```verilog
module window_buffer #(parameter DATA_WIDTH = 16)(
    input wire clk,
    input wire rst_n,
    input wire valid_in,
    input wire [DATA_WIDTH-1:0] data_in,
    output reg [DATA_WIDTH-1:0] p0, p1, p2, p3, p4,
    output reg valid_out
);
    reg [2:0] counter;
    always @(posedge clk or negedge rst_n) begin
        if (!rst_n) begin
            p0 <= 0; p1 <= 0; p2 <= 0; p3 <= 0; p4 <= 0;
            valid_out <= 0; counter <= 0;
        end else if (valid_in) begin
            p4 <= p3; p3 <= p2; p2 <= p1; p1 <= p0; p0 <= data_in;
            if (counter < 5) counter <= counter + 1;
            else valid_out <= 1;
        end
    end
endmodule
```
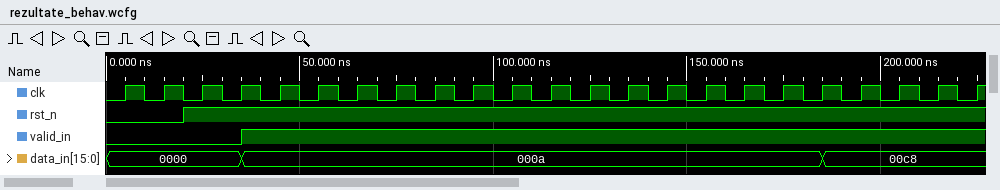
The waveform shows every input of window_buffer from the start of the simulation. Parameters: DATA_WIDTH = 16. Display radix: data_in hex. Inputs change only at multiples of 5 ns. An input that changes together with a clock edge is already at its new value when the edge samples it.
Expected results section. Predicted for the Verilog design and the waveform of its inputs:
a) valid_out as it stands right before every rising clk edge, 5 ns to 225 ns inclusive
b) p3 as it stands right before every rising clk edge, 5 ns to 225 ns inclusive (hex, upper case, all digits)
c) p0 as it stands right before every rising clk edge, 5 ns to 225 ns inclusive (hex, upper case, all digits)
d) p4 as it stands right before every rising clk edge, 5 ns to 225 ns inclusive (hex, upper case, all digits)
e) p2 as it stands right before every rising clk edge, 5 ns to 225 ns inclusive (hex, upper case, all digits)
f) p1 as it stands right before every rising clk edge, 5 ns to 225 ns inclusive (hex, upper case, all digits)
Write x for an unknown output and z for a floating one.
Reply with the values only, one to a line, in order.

0 0 0 0 0 0 0 0 0 1 1 1 1 1 1 1 1 1 1 1 1 1 1
0000, 0000, 0000, 0000, 0000, 0000, 0000, 000A, 000A, 000A, 000A, 000A, 000A, 000A, 000A, 000A, 000A, 000A, 000A, 000A, 000A, 000A, 00C8
0000, 0000, 0000, 0000, 000A, 000A, 000A, 000A, 000A, 000A, 000A, 000A, 000A, 000A, 000A, 000A, 000A, 000A, 000A, 00C8, 00C8, 00C8, 00C8
0000, 0000, 0000, 0000, 0000, 0000, 0000, 0000, 000A, 000A, 000A, 000A, 000A, 000A, 000A, 000A, 000A, 000A, 000A, 000A, 000A, 000A, 000A
0000, 0000, 0000, 0000, 0000, 0000, 000A, 000A, 000A, 000A, 000A, 000A, 000A, 000A, 000A, 000A, 000A, 000A, 000A, 000A, 000A, 00C8, 00C8
0000, 0000, 0000, 0000, 0000, 000A, 000A, 000A, 000A, 000A, 000A, 000A, 000A, 000A, 000A, 000A, 000A, 000A, 000A, 000A, 00C8, 00C8, 00C8
